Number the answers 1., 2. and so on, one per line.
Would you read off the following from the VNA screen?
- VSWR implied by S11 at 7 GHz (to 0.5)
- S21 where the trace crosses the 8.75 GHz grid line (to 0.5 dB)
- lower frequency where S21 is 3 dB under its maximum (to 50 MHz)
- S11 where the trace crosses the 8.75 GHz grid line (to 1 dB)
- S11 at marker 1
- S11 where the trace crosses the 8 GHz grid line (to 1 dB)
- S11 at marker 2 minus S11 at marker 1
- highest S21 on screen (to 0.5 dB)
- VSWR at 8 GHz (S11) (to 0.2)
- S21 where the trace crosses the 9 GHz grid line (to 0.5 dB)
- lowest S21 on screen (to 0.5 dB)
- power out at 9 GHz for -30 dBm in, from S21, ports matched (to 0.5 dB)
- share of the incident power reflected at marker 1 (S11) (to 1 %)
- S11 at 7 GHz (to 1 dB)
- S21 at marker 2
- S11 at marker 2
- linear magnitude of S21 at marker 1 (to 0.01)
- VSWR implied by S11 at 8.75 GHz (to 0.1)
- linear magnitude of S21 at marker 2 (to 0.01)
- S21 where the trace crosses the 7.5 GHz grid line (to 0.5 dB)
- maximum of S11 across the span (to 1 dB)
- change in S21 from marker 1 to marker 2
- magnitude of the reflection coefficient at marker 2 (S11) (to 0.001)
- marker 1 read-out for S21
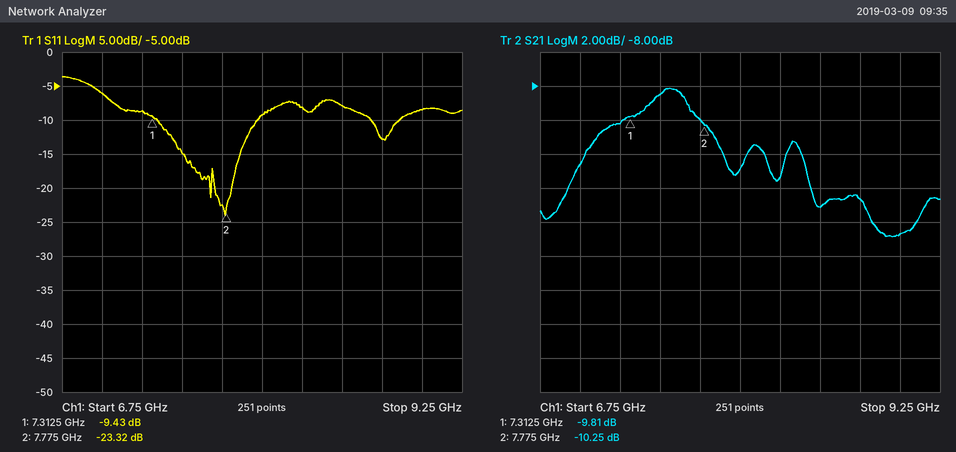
1. 3.0
2. -14.5 dB
3. 7.10 GHz
4. -13 dB
5. -9.43 dB
6. -9 dB
7. -13.89 dB
8. -8.0 dB
9. 2.0
10. -16.5 dB
11. -17.0 dB
12. -46.5 dBm
13. 11 %
14. -6 dB
15. -10.25 dB
16. -23.32 dB
17. 0.32
18. 1.6
19. 0.31
20. -8.5 dB
21. -4 dB
22. -0.44 dB
23. 0.068
24. -9.81 dB
